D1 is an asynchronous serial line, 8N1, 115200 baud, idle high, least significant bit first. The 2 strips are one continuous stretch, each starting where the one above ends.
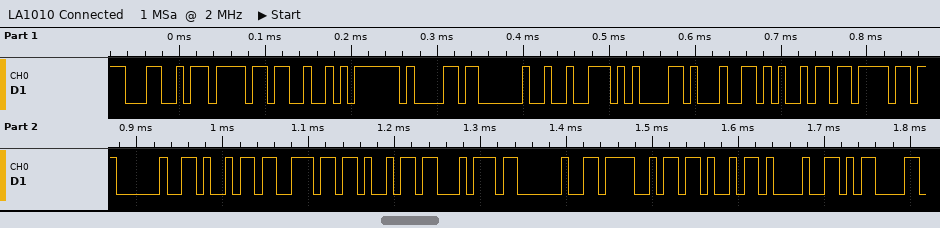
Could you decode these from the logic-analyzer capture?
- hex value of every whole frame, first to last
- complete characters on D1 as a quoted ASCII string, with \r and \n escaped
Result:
4C 6F 52 61 20 72 61 64 69 6F 20 69 6E 69 74 20 4F 4B 21 0D
"LoRa radio init OK!\r"
